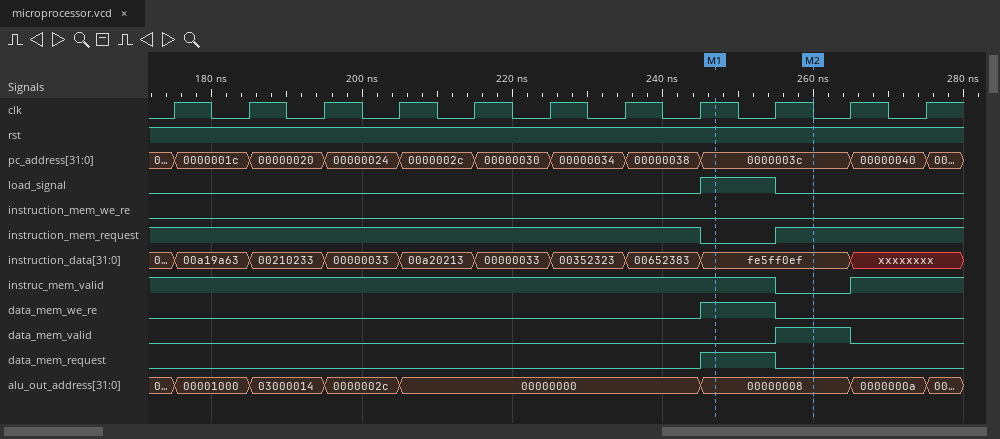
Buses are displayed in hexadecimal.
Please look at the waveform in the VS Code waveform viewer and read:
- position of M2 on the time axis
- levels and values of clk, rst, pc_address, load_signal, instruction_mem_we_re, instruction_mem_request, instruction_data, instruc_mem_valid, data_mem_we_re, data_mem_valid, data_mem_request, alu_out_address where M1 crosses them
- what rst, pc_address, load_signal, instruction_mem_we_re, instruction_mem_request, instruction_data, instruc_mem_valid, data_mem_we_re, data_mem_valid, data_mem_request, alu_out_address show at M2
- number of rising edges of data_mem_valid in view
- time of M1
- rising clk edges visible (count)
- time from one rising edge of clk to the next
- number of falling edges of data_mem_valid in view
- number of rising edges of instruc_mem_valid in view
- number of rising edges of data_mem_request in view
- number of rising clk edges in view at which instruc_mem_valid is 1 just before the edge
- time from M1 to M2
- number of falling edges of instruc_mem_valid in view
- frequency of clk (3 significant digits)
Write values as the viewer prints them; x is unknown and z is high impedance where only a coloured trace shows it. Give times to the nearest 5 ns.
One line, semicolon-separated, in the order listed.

260 ns; clk=1, rst=1, pc_address=0000003c, load_signal=1, instruction_mem_we_re=0, instruction_mem_request=0, instruction_data=fe5ff0ef, instruc_mem_valid=1, data_mem_we_re=1, data_mem_valid=0, data_mem_request=1, alu_out_address=00000008; rst=1, pc_address=0000003c, load_signal=0, instruction_mem_we_re=0, instruction_mem_request=1, instruction_data=fe5ff0ef, instruc_mem_valid=0, data_mem_we_re=0, data_mem_valid=1, data_mem_request=0, alu_out_address=00000008; 1; 245 ns; 11; 10 ns; 1; 1; 1; 10; 15 ns; 1; 100 MHz
